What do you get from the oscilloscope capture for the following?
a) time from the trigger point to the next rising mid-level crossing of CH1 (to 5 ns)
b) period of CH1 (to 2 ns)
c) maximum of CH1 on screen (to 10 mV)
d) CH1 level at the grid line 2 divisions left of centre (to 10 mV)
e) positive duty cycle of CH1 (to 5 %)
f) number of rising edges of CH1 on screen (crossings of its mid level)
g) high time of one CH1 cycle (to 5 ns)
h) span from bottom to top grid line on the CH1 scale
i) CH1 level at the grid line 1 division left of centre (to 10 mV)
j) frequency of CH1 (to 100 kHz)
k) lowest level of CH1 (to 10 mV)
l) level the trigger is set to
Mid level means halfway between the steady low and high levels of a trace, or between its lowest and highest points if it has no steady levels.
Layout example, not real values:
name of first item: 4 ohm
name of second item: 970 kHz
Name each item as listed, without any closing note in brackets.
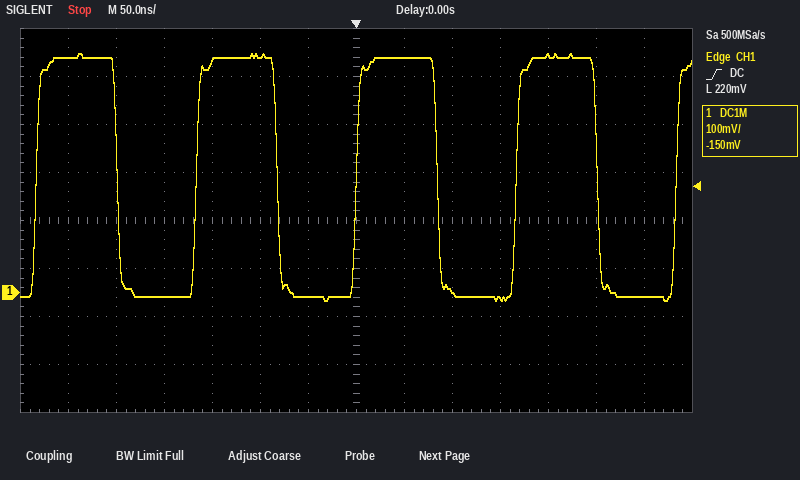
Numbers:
time from the trigger point to the next rising mid-level crossing of CH1: 165 ns
period of CH1: 166 ns
maximum of CH1 on screen: 500 mV
CH1 level at the grid line 2 divisions left of centre: 490 mV
positive duty cycle of CH1: 50 %
number of rising edges of CH1 on screen: 5
high time of one CH1 cycle: 85 ns
span from bottom to top grid line on the CH1 scale: 800 mV
CH1 level at the grid line 1 division left of centre: -10 mV
frequency of CH1: 6.0 MHz
lowest level of CH1: -20 mV
level the trigger is set to: 220 mV
